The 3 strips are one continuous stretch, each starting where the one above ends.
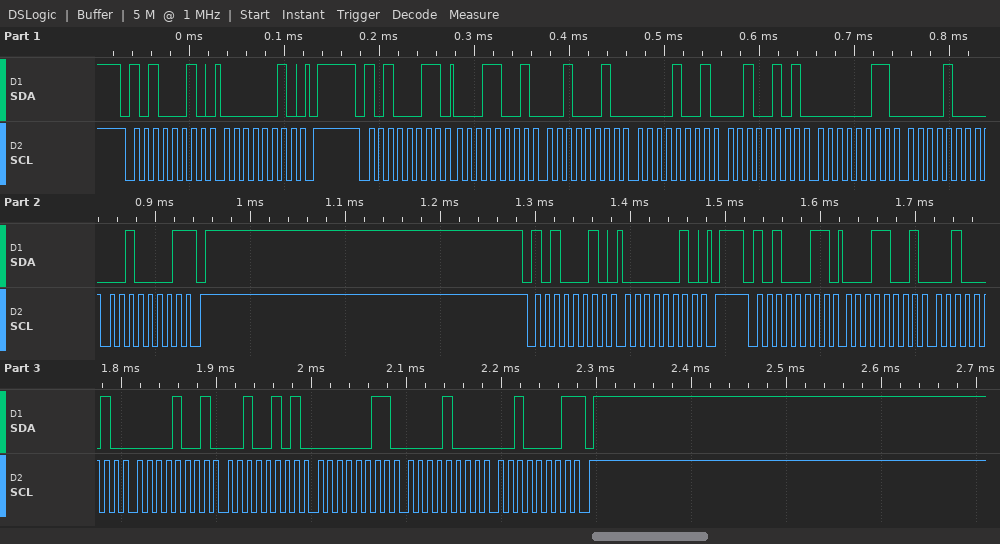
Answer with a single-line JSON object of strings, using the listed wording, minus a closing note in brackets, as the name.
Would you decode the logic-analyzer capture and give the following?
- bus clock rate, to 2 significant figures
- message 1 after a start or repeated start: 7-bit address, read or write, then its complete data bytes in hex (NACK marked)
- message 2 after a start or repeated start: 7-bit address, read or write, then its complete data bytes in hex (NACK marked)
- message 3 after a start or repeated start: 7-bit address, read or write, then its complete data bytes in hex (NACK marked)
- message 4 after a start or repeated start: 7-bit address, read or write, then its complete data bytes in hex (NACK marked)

{"bus clock rate, to 2 significant figures": "100 kHz", "message 1 after a start or repeated start: 7-bit address, read or write, then its complete data bytes in hex": "0x51 write: 02", "message 2 after a start or repeated start: 7-bit address, read or write, then its complete data bytes in hex": "0x51 read: 19 22 09 25 03 08 21 NACK", "message 3 after a start or repeated start: 7-bit address, read or write, then its complete data bytes in hex": "0x51 write: 02", "message 4 after a start or repeated start: 7-bit address, read or write, then its complete data bytes in hex": "0x51 read: 19 22 09 25 03 08 21 NACK"}
